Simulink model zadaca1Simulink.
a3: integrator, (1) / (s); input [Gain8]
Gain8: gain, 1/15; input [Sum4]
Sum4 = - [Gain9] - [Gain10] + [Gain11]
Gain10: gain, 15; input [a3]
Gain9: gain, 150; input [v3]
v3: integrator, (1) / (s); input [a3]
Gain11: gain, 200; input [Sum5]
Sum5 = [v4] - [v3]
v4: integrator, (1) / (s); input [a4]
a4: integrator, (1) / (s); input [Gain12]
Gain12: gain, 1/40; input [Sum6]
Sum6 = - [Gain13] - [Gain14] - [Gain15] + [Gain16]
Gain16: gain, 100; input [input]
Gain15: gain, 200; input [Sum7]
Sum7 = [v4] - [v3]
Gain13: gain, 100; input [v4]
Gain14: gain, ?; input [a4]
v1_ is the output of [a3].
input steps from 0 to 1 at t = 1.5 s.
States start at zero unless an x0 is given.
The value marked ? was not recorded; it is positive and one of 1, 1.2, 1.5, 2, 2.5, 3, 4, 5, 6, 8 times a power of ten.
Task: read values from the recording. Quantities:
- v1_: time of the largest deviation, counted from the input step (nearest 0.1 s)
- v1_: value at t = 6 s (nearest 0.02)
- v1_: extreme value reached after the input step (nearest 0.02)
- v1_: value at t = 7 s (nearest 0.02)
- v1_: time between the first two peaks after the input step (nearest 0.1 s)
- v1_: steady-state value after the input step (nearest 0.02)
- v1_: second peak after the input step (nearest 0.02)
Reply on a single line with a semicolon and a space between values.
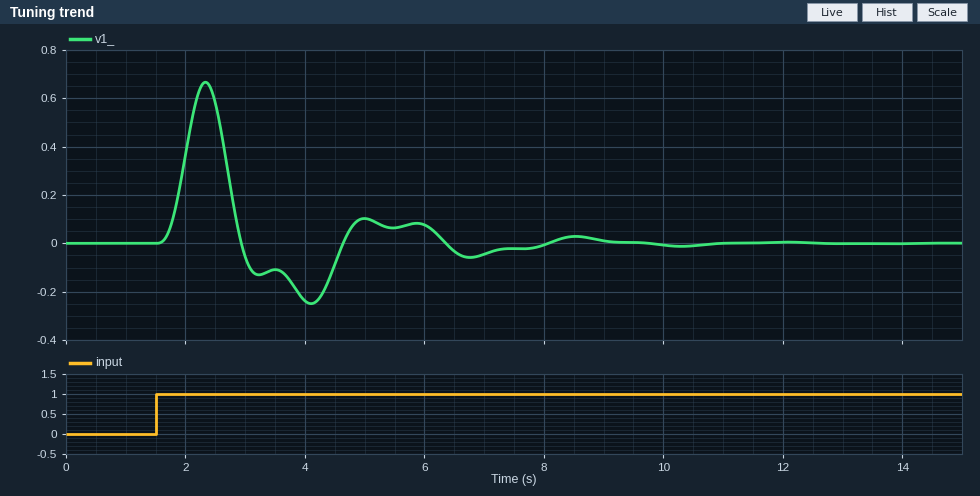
0.8 s; 0.08; 0.66; -0.04; 2.7 s; 0.00; 0.10
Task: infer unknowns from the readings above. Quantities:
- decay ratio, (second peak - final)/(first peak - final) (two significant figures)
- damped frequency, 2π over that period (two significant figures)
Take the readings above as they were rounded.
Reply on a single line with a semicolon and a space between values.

0.15; 2.3 rad/s
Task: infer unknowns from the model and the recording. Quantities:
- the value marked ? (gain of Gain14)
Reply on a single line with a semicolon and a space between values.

40
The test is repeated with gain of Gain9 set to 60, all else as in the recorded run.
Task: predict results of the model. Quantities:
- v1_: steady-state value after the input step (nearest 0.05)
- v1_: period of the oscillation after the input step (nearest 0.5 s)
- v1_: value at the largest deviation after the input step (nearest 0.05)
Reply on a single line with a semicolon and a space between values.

0.00; 4.0 s; 0.90
